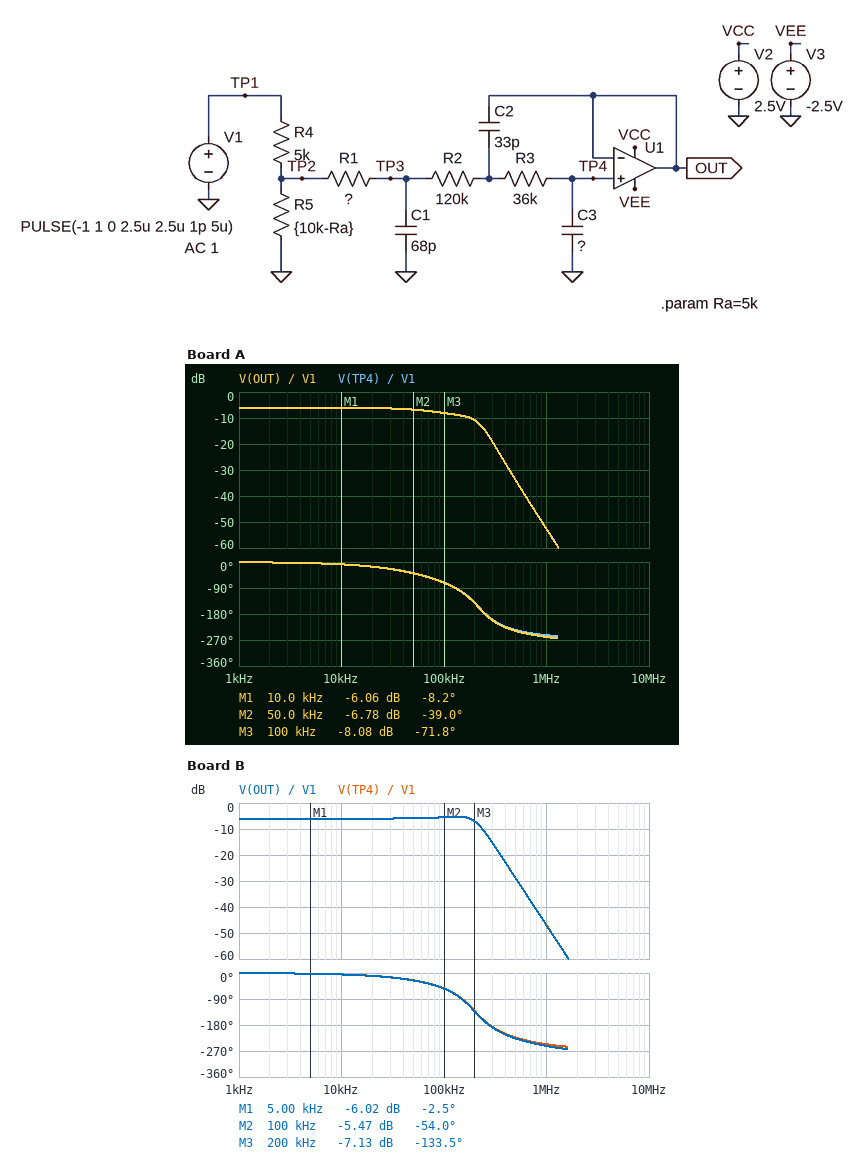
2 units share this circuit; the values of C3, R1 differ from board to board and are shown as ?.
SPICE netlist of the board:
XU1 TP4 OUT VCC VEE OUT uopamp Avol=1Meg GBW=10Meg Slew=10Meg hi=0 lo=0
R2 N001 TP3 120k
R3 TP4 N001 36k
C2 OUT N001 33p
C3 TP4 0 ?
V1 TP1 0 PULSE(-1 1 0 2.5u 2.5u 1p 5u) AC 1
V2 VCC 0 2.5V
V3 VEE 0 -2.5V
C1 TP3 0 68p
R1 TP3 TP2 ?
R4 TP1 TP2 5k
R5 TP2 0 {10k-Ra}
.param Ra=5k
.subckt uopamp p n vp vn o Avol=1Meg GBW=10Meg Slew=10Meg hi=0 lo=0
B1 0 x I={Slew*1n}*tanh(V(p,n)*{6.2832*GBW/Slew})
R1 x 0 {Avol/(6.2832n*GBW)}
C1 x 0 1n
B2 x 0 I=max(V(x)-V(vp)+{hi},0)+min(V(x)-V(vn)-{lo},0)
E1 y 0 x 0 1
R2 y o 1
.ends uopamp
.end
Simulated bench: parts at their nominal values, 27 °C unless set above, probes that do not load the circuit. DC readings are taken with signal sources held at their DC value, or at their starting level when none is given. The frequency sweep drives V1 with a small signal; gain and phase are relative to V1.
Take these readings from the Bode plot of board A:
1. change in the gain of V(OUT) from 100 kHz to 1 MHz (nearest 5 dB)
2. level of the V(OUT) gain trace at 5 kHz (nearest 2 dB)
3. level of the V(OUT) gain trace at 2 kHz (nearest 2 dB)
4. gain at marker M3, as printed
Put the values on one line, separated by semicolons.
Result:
-45 dB; -6 dB; -6 dB; -8.08 dB
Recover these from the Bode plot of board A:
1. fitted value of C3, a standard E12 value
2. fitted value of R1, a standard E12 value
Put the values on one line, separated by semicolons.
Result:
3.3 pF; 22 kΩ
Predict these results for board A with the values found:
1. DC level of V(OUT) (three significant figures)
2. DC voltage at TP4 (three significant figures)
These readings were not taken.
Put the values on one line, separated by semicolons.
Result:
-500 mV; -500 mV
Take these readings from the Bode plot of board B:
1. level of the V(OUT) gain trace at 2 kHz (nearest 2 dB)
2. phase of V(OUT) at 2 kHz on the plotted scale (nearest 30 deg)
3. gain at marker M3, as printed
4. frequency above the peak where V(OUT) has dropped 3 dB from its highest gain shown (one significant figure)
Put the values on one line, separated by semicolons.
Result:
-6 dB; 0 deg; -7.13 dB; 200 kHz
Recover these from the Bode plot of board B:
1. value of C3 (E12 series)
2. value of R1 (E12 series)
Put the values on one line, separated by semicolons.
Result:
3.9 pF; 8.2 kΩ
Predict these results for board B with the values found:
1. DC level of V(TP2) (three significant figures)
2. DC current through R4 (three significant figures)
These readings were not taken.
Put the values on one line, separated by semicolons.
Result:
-500 mV; 100 µA
